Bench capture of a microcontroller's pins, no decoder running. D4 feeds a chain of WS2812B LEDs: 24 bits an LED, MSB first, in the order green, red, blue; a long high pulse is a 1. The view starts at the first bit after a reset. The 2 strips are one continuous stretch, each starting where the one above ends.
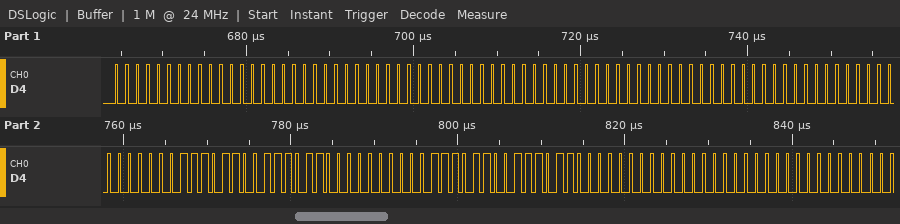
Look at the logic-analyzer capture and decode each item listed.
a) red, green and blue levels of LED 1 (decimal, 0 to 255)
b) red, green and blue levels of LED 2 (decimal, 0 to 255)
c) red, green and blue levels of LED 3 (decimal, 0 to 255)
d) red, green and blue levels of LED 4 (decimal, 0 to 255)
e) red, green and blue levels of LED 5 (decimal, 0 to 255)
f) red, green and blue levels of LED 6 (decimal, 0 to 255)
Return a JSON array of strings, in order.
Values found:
["0, 0, 0", "0, 0, 0", "0, 0, 0", "59, 0, 59", "59, 0, 59", "0, 0, 0"]
